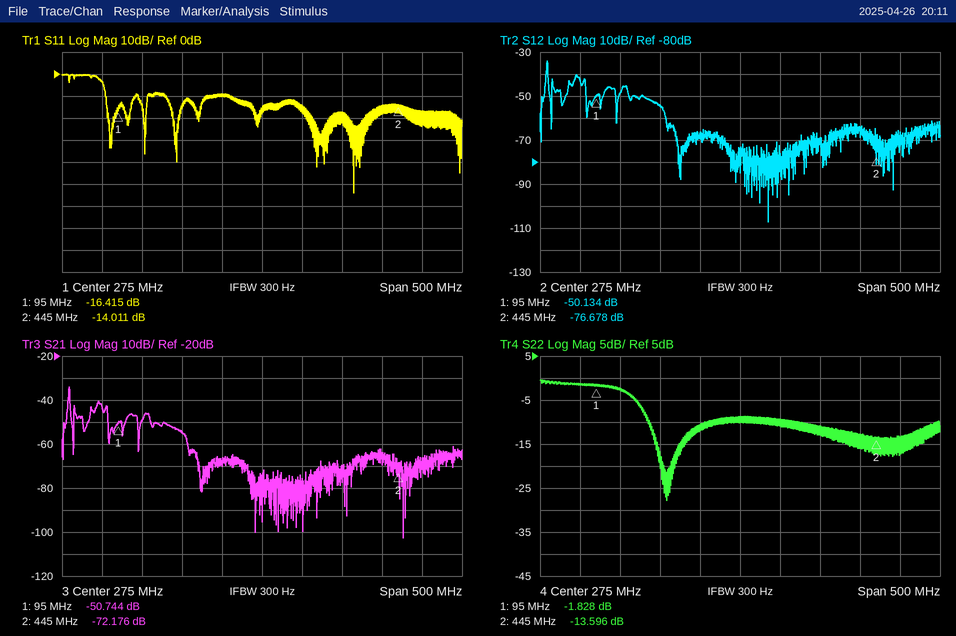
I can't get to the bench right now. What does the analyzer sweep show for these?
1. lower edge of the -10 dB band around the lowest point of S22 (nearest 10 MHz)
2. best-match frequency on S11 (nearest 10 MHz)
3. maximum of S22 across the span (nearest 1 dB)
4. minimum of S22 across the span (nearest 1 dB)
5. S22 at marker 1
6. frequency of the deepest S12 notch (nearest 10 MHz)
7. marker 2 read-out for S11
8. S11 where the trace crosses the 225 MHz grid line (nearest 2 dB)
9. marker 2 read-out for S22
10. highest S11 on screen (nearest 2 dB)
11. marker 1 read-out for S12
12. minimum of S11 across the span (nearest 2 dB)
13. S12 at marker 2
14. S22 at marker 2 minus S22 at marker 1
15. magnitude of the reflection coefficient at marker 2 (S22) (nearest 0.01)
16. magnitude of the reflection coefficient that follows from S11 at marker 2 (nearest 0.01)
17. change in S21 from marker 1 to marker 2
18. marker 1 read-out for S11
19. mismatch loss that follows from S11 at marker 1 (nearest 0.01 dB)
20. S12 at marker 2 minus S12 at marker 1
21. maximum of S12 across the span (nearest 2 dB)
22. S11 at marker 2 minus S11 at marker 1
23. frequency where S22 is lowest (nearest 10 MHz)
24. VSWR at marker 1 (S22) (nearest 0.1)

160 MHz
390 MHz
0 dB
-28 dB
-1.828 dB
310 MHz
-14.011 dB
-10 dB
-13.596 dB
0 dB
-50.134 dB
-54 dB
-76.678 dB
-11.768 dB
0.21
0.20
-21.432 dB
-16.415 dB
0.10 dB
-26.544 dB
-34 dB
2.404 dB
180 MHz
9.5
